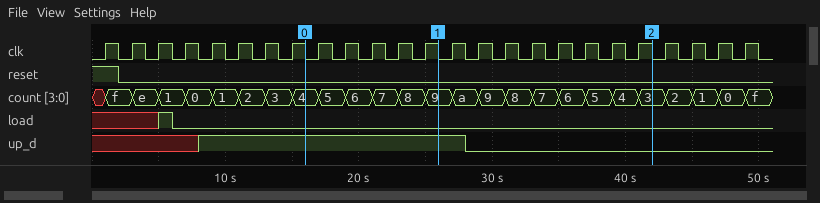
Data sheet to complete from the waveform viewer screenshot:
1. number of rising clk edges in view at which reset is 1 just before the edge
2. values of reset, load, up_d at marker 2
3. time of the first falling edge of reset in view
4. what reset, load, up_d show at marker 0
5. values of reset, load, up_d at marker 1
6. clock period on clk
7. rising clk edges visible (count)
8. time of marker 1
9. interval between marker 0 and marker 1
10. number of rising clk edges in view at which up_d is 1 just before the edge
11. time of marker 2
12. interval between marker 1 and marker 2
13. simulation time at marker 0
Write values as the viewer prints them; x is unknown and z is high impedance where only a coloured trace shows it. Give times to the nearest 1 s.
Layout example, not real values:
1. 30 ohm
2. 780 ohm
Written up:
1. 1
2. reset=0, load=0, up_d=0
3. 2 s
4. reset=0, load=0, up_d=1
5. reset=0, load=0, up_d=1
6. 2 s
7. 25
8. 26 s
9. 10 s
10. 10
11. 42 s
12. 16 s
13. 16 s
